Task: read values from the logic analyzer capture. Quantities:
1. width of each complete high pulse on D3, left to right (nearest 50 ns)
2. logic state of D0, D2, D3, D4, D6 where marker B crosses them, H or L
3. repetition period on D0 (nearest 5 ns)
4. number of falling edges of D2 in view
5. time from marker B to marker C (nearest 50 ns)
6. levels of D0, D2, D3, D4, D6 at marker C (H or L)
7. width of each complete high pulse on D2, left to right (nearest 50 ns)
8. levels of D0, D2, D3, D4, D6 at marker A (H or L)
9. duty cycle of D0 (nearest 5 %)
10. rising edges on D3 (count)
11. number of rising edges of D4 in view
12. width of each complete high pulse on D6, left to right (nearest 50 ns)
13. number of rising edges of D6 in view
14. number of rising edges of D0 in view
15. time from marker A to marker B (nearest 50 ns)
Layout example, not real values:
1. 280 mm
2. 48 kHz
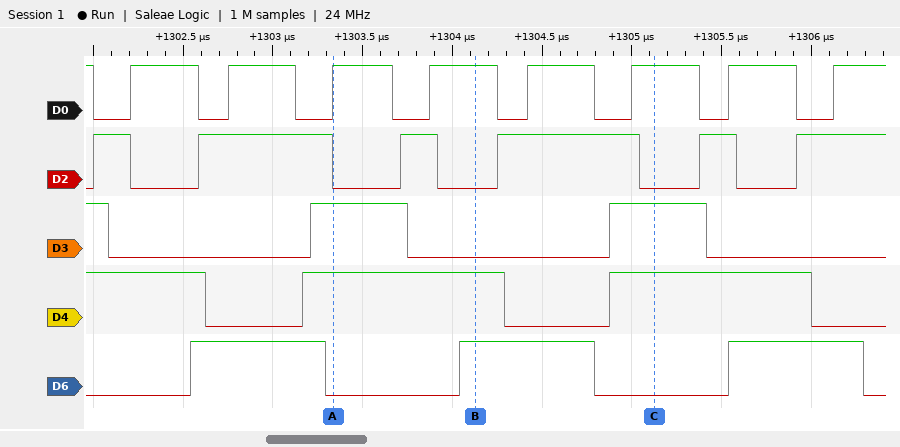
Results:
1. 550 ns, 550 ns
2. D0=H, D2=L, D3=L, D4=H, D6=H
3. 560 ns
4. 5
5. 1000 ns
6. D0=H, D2=L, D3=H, D4=H, D6=L
7. 200 ns, 750 ns, 200 ns, 800 ns, 200 ns
8. D0=H, D2=L, D3=H, D4=H, D6=L
9. 65 %
10. 2
11. 2
12. 750 ns, 750 ns, 750 ns
13. 3
14. 8
15. 800 ns
